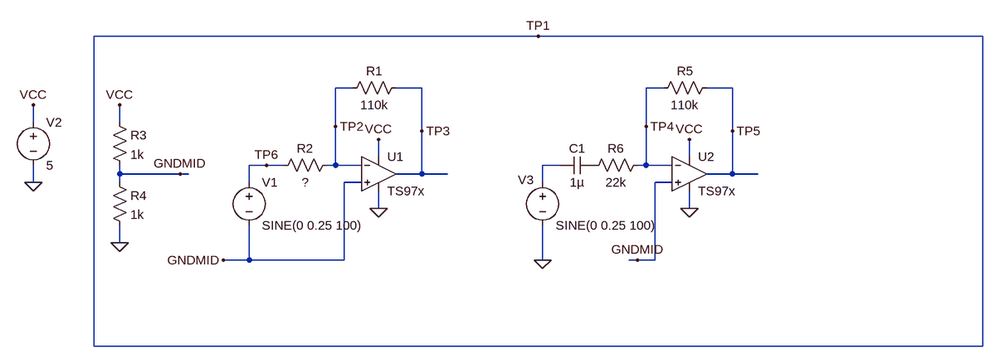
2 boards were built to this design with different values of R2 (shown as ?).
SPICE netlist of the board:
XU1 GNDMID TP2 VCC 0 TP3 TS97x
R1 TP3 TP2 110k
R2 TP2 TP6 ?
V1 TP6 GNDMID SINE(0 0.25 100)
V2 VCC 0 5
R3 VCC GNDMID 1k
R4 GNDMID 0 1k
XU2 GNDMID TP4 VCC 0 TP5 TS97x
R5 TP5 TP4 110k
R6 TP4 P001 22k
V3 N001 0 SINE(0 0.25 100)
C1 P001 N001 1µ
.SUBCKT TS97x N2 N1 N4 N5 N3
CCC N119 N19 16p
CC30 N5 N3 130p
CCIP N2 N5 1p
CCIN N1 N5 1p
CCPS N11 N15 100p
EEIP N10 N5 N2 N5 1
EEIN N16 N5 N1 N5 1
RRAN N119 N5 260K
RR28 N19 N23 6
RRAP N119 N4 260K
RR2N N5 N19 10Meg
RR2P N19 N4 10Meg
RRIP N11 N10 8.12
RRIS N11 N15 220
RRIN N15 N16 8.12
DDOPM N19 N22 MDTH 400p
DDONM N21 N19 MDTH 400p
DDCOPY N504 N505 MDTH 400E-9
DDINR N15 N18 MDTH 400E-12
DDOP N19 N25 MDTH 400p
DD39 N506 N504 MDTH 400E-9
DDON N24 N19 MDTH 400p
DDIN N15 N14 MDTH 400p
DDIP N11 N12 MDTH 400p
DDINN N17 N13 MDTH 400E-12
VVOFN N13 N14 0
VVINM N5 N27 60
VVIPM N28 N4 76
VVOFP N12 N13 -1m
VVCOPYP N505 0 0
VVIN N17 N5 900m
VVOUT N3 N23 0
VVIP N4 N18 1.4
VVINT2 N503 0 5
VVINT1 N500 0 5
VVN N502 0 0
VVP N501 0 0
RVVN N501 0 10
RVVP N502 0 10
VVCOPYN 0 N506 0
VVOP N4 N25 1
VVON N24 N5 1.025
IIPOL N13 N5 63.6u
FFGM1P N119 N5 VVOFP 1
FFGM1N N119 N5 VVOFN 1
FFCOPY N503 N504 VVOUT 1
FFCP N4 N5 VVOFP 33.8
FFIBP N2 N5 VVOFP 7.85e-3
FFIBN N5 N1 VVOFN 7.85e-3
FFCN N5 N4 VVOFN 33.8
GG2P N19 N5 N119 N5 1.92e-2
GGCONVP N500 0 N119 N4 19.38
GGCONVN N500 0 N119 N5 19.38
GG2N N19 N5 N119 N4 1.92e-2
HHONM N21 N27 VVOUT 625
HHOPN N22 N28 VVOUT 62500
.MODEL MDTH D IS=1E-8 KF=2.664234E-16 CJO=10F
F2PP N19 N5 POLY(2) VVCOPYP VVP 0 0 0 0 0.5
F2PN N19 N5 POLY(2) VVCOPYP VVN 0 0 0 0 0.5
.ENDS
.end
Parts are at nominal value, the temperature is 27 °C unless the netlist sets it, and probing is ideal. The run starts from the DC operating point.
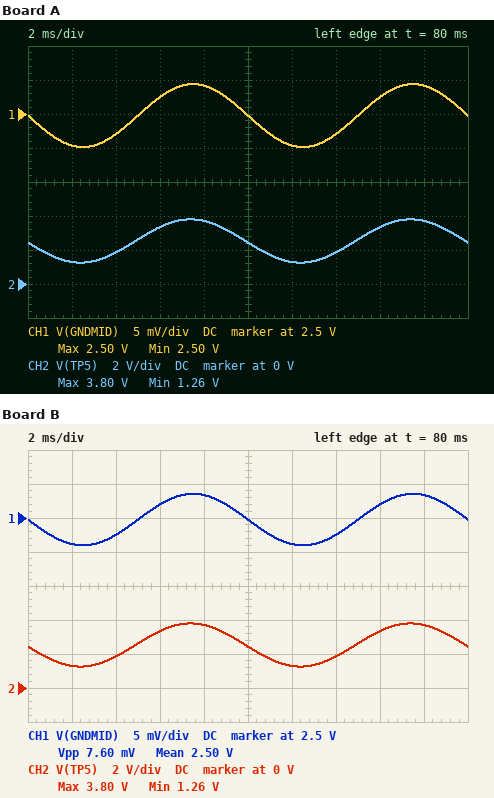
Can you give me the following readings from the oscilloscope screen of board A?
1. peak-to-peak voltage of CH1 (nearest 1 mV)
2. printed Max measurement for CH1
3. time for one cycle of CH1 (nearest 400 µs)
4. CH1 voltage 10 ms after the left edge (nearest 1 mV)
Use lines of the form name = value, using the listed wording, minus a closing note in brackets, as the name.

peak-to-peak voltage of CH1 = 9 mV
printed Max measurement for CH1 = 2.50 V
time for one cycle of CH1 = 10.0 ms
CH1 voltage 10 ms after the left edge = 2.500 V
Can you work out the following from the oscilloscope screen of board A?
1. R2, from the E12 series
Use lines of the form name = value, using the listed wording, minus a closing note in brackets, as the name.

R2, from the E12 series = 27 kΩ
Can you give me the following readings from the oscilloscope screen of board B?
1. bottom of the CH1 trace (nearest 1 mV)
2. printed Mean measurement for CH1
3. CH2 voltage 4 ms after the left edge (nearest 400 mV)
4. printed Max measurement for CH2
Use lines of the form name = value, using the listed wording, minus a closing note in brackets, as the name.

bottom of the CH1 trace = 2.496 V
printed Mean measurement for CH1 = 2.50 V
CH2 voltage 4 ms after the left edge = 2.0 V
printed Max measurement for CH2 = 3.80 V
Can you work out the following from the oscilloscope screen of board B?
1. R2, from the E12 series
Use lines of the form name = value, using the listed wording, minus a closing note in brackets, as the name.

R2, from the E12 series = 33 kΩ
